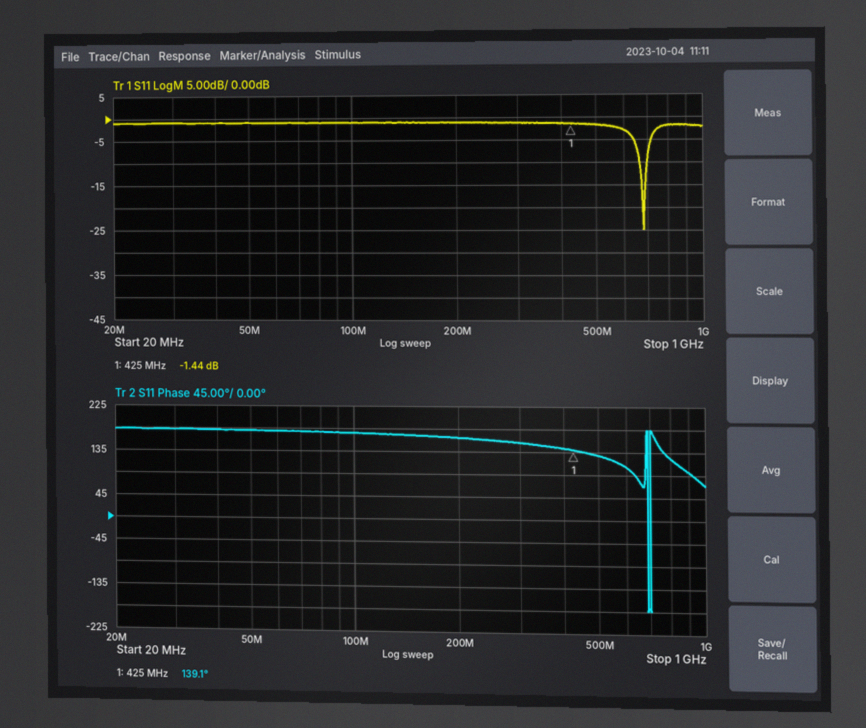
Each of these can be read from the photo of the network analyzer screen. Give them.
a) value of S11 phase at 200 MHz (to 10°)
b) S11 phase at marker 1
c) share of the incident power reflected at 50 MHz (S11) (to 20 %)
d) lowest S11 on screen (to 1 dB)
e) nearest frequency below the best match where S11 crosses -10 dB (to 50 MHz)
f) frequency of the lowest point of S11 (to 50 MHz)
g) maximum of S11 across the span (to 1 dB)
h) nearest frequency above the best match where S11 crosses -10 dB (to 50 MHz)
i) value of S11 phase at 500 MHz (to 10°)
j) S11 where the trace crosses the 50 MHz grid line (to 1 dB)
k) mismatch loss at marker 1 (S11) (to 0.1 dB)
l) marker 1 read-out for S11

160°
139.1°
80 %
-25 dB
650 MHz
700 MHz
-1 dB
700 MHz
130°
-1 dB
5.5 dB
-1.44 dB
